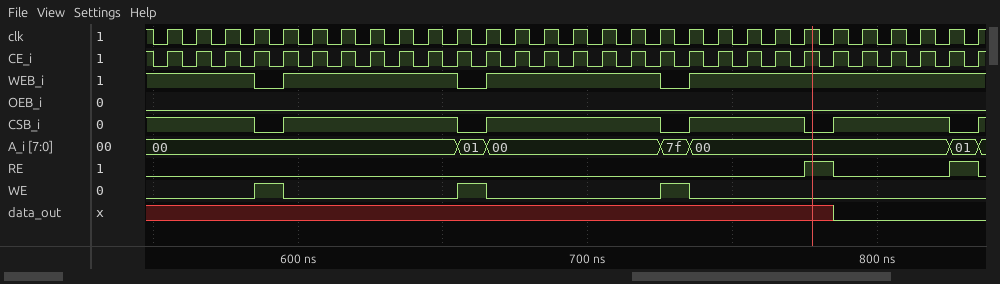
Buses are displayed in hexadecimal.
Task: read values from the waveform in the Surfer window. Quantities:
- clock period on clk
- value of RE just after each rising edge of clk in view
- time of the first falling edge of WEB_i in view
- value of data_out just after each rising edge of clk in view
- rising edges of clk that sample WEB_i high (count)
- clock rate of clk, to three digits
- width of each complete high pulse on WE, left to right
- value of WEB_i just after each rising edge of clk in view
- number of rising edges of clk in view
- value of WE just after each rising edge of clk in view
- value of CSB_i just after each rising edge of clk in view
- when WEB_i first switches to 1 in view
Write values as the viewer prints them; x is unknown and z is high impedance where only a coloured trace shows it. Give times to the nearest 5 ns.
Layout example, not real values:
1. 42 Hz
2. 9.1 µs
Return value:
1. 10 ns
2. 0 0 0 0 0 0 0 0 0 0 0 0 0 0 0 0 0 0 0 0 0 0 1 0 0 0 0 1 0
3. 585 ns
4. x x x x x x x x x x x x x x x x x x x x x x x 0 0 0 0 0 0
5. 26
6. 100 MHz
7. 10 ns, 10 ns, 10 ns
8. 1 1 1 0 1 1 1 1 1 1 0 1 1 1 1 1 1 0 1 1 1 1 1 1 1 1 1 1 1
9. 29
10. 0 0 0 1 0 0 0 0 0 0 1 0 0 0 0 0 0 1 0 0 0 0 0 0 0 0 0 0 0
11. 1 1 1 0 1 1 1 1 1 1 0 1 1 1 1 1 1 0 1 1 1 1 0 1 1 1 1 0 1
12. 595 ns
